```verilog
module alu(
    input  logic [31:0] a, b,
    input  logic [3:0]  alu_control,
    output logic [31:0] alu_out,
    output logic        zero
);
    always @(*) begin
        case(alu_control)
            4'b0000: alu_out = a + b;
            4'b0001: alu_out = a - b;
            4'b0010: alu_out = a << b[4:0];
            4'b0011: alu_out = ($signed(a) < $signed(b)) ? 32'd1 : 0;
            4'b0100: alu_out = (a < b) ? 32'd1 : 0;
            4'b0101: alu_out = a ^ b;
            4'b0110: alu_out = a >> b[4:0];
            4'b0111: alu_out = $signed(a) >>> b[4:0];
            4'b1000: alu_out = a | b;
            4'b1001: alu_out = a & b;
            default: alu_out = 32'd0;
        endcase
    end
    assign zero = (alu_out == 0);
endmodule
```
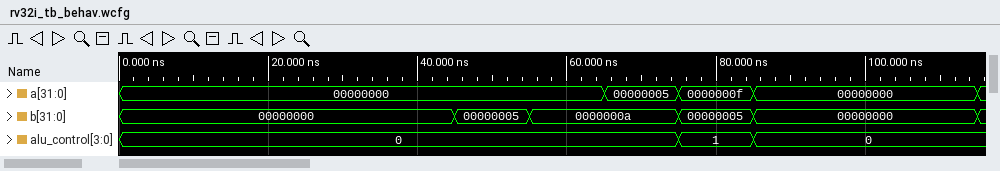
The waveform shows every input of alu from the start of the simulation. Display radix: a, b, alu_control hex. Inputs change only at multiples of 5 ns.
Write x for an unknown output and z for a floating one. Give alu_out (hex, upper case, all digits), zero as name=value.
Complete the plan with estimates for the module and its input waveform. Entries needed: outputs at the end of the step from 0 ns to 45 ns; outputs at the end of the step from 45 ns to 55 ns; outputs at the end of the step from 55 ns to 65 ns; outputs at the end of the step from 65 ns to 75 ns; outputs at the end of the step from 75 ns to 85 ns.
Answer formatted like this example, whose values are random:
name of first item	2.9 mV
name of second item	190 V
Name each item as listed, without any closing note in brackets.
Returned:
outputs at the end of the step from 0 ns to 45 ns	alu_out=00000000, zero=1
outputs at the end of the step from 45 ns to 55 ns	alu_out=00000005, zero=0
outputs at the end of the step from 55 ns to 65 ns	alu_out=0000000A, zero=0
outputs at the end of the step from 65 ns to 75 ns	alu_out=0000000F, zero=0
outputs at the end of the step from 75 ns to 85 ns	alu_out=0000000A, zero=0
